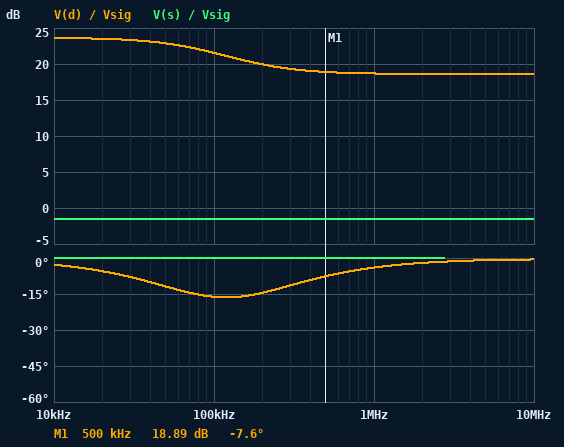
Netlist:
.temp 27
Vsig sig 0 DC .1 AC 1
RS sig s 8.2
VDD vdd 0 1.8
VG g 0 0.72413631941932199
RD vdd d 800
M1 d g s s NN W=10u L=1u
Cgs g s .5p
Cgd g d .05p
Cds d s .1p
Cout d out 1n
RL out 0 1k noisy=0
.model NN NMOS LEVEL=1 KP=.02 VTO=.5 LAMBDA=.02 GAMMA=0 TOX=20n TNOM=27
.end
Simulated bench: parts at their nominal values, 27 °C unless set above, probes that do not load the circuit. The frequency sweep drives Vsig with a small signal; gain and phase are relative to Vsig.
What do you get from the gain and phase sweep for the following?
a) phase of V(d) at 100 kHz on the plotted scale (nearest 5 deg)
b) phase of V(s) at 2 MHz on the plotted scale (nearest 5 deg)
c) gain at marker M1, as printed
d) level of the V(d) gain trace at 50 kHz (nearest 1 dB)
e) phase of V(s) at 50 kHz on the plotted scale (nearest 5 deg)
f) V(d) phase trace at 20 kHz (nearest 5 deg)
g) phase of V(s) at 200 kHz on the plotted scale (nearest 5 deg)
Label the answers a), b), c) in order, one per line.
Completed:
a) -15 deg
b) 0 deg
c) 18.89 dB
d) 23 dB
e) 0 deg
f) -5 deg
g) 0 deg
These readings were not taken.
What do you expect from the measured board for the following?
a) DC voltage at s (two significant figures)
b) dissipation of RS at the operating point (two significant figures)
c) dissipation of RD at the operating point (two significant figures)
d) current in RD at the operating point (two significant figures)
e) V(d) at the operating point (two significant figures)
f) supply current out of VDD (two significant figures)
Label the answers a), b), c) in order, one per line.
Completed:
a) 110 mV
b) 14 µW
c) 1.4 mW
d) 1.3 mA
e) 760 mV
f) 1.3 mA
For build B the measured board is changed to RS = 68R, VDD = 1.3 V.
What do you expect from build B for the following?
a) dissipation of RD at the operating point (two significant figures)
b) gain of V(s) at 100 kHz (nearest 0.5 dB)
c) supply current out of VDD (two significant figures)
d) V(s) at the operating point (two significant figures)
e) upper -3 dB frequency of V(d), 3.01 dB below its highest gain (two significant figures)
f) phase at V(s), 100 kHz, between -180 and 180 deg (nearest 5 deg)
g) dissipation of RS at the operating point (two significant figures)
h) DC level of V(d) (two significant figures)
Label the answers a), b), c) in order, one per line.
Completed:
a) 340 µW
b) -6.5 dB
c) 650 µA
d) 140 mV
e) 140 kHz
f) 0 deg
g) 29 µW
h) 780 mV
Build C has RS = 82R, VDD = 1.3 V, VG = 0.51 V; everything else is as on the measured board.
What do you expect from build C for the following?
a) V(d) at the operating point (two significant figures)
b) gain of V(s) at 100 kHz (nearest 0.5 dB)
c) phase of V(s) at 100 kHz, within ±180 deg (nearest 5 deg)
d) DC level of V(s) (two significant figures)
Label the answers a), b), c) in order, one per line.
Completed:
a) 1.3 V
b) 0 dB
c) 0 deg
d) 100 mV
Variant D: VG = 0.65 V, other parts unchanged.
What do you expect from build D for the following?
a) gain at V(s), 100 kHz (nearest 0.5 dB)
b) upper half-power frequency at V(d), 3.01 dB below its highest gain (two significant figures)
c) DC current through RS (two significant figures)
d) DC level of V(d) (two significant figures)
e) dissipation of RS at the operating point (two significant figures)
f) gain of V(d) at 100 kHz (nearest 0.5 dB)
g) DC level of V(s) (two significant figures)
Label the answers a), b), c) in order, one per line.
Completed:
a) -0.5 dB
b) 140 kHz
c) 240 µA
d) 1.6 V
e) 460 nW
f) 15.0 dB
g) 100 mV
